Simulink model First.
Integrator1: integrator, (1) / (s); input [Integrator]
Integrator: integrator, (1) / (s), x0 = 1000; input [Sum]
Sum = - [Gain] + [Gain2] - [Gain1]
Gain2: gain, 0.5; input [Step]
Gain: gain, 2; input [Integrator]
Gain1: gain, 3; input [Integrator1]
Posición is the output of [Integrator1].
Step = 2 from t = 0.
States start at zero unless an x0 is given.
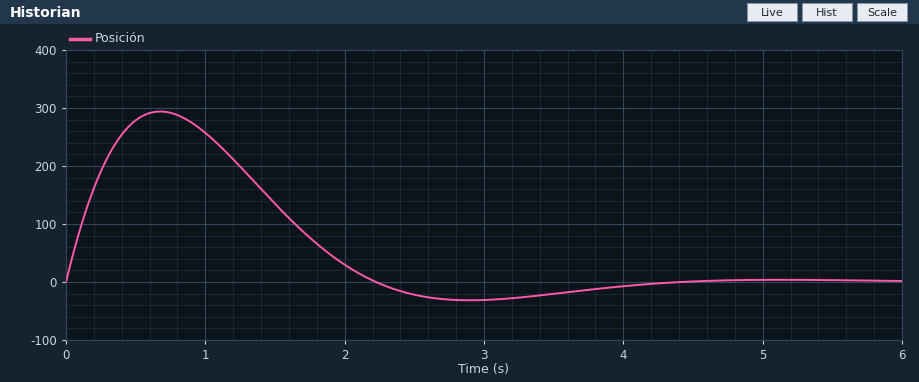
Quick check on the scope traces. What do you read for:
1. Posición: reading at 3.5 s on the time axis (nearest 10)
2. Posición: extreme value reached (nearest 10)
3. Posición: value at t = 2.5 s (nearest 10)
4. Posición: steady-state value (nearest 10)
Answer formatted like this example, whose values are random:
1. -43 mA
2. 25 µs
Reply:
1. -20
2. 290
3. -20
4. 0
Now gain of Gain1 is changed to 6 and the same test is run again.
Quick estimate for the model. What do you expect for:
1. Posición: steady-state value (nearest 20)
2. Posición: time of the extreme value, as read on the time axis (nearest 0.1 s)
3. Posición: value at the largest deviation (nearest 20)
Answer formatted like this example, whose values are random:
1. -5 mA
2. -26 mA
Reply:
1. 0
2. 0.5 s
3. 240
